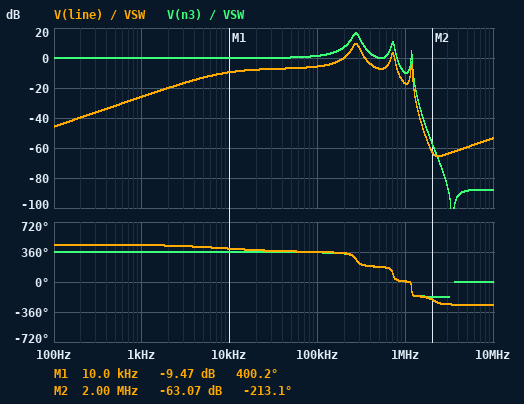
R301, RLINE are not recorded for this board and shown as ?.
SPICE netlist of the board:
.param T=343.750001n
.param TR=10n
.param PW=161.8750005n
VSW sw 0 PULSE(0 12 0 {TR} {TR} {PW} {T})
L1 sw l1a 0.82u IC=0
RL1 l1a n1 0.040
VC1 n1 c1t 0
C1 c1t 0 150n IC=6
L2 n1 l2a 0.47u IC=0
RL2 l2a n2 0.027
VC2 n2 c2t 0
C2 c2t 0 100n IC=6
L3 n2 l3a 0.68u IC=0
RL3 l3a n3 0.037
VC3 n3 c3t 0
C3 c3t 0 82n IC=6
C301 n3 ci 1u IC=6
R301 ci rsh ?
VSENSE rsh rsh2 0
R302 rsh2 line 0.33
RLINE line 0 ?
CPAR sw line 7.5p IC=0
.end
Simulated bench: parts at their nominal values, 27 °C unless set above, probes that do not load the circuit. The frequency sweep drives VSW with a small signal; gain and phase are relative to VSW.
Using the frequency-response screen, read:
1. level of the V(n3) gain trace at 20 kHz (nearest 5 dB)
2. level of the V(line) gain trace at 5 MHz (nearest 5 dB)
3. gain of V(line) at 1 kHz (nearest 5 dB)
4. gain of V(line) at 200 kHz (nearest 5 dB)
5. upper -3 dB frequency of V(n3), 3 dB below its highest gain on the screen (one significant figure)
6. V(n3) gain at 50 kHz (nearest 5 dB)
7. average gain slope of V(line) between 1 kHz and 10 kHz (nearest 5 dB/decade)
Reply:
0 dB
-60 dB
-25 dB
0 dB
300 kHz
0 dB
15 dB/decade
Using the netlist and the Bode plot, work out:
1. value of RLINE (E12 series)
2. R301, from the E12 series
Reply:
8.2 Ω
10 Ω
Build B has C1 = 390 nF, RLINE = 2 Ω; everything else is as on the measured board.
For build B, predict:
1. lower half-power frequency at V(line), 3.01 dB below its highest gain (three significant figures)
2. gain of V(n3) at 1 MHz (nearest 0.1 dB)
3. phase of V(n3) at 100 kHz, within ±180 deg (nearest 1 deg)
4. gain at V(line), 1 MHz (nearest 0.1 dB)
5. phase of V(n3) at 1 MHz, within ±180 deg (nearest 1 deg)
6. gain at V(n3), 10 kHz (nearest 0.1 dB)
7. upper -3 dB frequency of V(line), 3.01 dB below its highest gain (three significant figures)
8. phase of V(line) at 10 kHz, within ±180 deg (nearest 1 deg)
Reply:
201 kHz
-17.0 dB
-8 deg
-32.8 dB
-1 deg
0 dB
244 kHz
52 deg
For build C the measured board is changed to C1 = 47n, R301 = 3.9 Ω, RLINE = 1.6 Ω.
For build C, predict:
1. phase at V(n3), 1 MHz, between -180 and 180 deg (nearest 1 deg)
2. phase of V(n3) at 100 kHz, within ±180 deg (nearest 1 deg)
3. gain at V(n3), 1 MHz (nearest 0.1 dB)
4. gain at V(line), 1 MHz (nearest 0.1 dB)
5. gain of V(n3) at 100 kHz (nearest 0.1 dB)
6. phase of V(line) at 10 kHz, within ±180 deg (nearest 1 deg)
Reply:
45 deg
-14 deg
-6.5 dB
-17.8 dB
1.3 dB
69 deg
